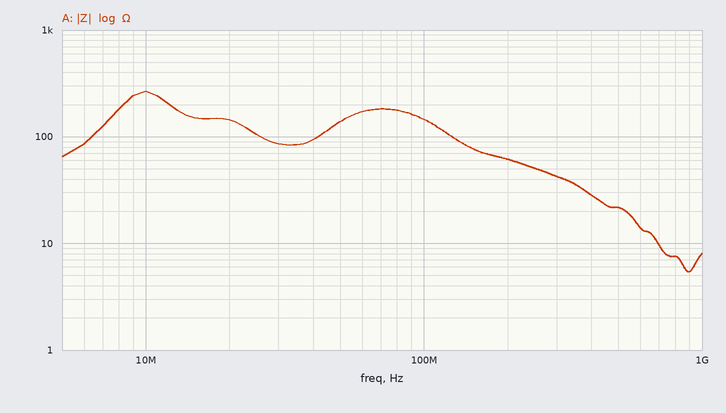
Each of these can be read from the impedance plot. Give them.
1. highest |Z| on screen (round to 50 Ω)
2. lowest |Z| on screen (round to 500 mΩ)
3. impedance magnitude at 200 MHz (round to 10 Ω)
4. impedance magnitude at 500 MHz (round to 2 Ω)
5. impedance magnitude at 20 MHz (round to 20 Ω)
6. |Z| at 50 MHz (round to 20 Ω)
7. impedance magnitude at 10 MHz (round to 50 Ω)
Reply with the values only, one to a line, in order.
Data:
250 Ω
5.5 Ω
60 Ω
22 Ω
140 Ω
140 Ω
250 Ω
